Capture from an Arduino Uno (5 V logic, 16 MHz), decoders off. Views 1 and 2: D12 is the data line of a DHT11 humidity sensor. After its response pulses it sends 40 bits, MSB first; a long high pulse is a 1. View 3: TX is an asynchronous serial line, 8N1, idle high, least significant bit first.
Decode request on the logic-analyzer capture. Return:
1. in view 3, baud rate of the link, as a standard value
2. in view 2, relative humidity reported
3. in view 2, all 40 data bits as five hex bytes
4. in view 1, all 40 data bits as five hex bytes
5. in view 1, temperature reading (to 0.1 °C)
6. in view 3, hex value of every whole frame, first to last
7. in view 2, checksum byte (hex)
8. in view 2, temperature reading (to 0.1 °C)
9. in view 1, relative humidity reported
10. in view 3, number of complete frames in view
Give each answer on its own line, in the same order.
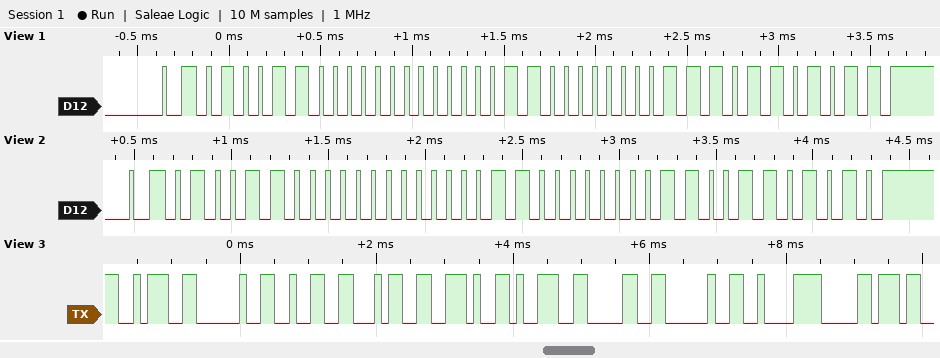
9600 baud
76 %
4C 00 18 06 6A
4C 00 18 07 6B
24.7 °C
0x3A 0x20 0x32 0x34 0x2E 0x39 0x30 0x20 0xC2 0xB0
0x6A
24.6 °C
76 %
10
